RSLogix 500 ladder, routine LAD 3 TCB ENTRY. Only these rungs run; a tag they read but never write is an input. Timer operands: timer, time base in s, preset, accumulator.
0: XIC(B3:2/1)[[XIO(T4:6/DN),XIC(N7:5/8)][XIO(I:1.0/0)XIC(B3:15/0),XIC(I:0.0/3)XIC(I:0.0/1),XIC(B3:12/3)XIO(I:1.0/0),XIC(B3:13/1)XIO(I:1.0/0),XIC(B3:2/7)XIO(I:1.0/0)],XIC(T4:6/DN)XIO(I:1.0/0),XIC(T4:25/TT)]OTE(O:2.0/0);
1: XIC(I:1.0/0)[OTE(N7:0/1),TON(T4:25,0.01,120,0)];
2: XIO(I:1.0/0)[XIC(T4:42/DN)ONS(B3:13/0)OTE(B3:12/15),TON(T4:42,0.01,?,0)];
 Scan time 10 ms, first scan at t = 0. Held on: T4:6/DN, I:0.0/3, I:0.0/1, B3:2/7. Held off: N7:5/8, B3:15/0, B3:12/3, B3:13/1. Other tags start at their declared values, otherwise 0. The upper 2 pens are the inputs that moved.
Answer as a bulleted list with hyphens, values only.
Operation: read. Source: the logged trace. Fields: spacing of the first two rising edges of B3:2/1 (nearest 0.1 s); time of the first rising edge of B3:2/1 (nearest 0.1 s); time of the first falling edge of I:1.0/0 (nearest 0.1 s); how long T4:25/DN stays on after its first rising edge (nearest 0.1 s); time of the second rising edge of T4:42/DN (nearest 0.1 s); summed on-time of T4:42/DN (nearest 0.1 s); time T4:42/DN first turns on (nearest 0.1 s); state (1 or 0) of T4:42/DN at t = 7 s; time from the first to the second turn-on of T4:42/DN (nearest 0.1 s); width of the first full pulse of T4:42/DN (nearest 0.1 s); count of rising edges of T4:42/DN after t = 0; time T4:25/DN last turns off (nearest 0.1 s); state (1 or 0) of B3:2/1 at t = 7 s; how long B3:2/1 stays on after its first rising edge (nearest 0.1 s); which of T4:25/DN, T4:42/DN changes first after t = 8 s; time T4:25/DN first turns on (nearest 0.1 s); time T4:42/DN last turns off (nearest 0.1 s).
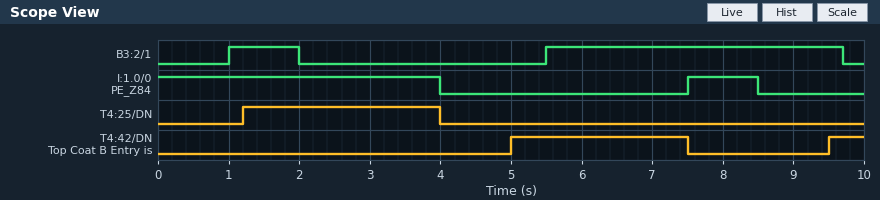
- 4.5 s
- 1.0 s
- 4.0 s
- 2.8 s
- 9.5 s
- 3.0 s
- 5.0 s
- 1
- 4.5 s
- 2.5 s
- 2
- 4.0 s
- 1
- 1.0 s
- T4:42/DN
- 1.2 s
- 7.5 s
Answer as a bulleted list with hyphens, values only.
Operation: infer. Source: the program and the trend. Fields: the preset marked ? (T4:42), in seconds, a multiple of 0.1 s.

- 1.0 s
